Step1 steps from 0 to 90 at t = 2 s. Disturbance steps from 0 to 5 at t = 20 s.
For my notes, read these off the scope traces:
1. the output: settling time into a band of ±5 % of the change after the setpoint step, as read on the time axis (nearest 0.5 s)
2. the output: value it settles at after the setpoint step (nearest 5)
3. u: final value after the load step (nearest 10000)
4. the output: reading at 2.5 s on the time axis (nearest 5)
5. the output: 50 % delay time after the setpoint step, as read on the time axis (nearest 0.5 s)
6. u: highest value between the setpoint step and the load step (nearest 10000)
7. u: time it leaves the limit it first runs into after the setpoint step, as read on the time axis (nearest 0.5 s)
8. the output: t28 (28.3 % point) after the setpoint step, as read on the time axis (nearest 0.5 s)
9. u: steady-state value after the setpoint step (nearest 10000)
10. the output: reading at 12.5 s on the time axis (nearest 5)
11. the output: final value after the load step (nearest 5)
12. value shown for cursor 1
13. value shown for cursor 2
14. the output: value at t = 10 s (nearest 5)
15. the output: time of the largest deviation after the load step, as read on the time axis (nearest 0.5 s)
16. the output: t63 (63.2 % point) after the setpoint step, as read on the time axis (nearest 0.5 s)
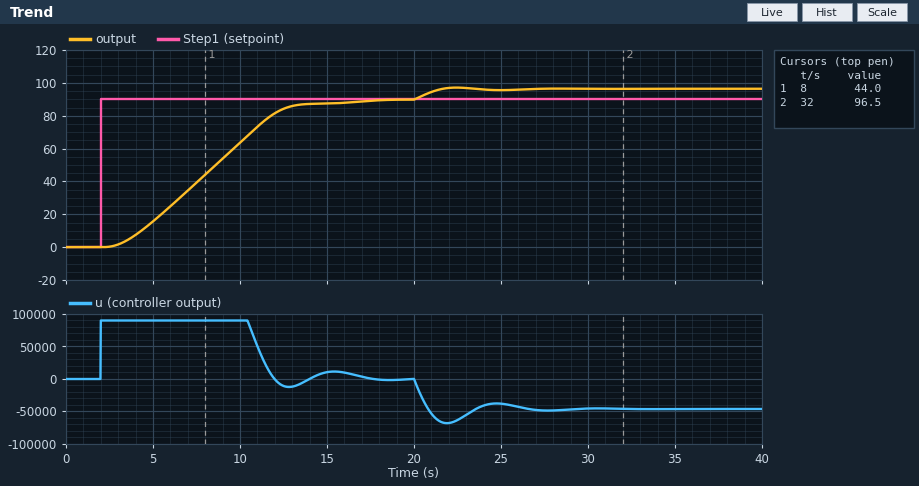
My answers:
13.0 s
90
-50000
0
8.0 s
90000
10.5 s
6.0 s
0
85
95
44.0
96.5
65
22.5 s
9.5 s
